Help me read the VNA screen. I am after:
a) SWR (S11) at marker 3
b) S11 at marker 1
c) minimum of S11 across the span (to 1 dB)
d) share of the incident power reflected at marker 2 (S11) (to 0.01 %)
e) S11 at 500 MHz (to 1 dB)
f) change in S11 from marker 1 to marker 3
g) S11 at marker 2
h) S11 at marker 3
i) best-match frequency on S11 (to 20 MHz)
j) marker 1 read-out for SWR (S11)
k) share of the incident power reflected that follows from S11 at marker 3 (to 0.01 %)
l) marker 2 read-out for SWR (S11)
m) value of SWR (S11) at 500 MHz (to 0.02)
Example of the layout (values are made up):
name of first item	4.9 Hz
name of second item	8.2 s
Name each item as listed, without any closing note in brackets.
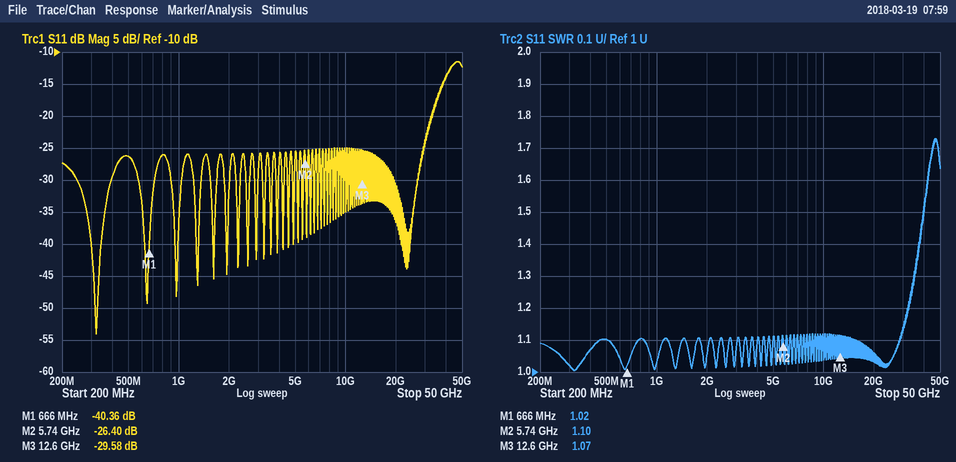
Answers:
SWR (S11) at marker 3	1.07
S11 at marker 1	-40.36 dB
minimum of S11 across the span	-54 dB
share of the incident power reflected at marker 2 (S11)	0.23 %
S11 at 500 MHz	-26 dB
change in S11 from marker 1 to marker 3	10.78 dB
S11 at marker 2	-26.40 dB
S11 at marker 3	-29.58 dB
best-match frequency on S11	320 MHz
marker 1 read-out for SWR	1.02
share of the incident power reflected that follows from S11 at marker 3	0.11 %
marker 2 read-out for SWR	1.10
value of SWR (S11) at 500 MHz	1.10
